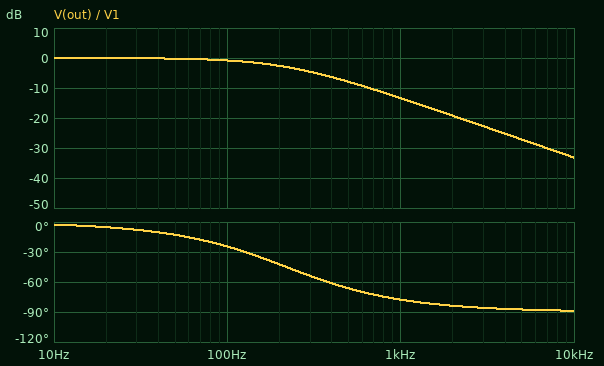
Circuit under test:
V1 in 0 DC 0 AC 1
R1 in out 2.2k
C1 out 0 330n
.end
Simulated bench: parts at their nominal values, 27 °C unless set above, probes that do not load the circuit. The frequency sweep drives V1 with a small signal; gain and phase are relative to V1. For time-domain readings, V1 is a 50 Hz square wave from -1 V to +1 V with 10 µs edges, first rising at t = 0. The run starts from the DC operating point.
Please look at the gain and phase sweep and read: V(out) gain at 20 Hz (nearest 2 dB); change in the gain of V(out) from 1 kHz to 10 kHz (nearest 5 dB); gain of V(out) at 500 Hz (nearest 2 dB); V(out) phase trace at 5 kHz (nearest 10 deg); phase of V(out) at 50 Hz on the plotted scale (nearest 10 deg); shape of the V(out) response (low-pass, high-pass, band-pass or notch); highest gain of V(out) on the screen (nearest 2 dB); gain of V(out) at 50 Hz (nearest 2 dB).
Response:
0 dB
-20 dB
-8 dB
-90 deg
-10 deg
low-pass
0 dB
0 dB
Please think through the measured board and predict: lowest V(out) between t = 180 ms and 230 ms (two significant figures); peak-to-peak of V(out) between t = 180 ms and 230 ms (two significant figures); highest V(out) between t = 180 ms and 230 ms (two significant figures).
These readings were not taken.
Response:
-1.0 V
2.0 V
1.0 V
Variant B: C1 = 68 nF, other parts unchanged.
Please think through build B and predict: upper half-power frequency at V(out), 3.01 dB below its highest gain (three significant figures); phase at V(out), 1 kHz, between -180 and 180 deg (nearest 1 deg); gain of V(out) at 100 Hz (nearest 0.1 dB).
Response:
1.06 kHz
-43 deg
0 dB
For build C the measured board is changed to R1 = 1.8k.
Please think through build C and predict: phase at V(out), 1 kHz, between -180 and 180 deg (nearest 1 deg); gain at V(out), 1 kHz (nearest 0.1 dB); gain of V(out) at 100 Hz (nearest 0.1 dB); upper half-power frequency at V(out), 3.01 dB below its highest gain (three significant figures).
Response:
-75 deg
-11.7 dB
-0.6 dB
268 Hz
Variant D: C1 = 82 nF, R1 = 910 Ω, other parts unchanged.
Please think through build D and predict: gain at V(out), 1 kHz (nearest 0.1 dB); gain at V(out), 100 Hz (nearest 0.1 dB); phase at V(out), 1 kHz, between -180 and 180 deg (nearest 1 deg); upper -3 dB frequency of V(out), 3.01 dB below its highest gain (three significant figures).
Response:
-0.9 dB
0 dB
-25 deg
2.13 kHz
